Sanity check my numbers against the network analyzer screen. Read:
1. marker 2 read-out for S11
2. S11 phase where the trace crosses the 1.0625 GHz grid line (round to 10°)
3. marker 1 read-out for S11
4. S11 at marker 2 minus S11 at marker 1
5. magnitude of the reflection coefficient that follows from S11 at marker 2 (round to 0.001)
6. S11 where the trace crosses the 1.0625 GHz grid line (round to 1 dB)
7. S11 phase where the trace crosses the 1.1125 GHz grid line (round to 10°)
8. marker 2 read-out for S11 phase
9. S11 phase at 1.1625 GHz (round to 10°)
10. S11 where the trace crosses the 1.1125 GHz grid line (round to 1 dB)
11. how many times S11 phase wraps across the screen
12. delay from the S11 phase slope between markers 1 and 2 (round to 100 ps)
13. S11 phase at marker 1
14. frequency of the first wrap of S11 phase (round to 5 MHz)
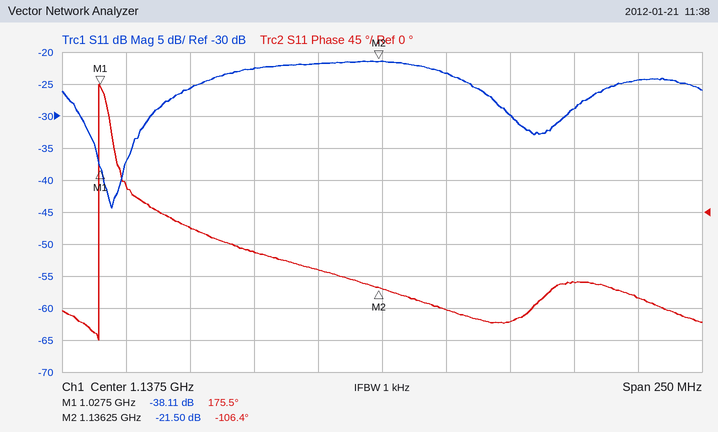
-21.50 dB
-20°
-38.11 dB
16.61 dB
0.084
-26 dB
-80°
-106.4°
-140°
-22 dB
1
7.2 ns
175.5°
1.025 GHz
